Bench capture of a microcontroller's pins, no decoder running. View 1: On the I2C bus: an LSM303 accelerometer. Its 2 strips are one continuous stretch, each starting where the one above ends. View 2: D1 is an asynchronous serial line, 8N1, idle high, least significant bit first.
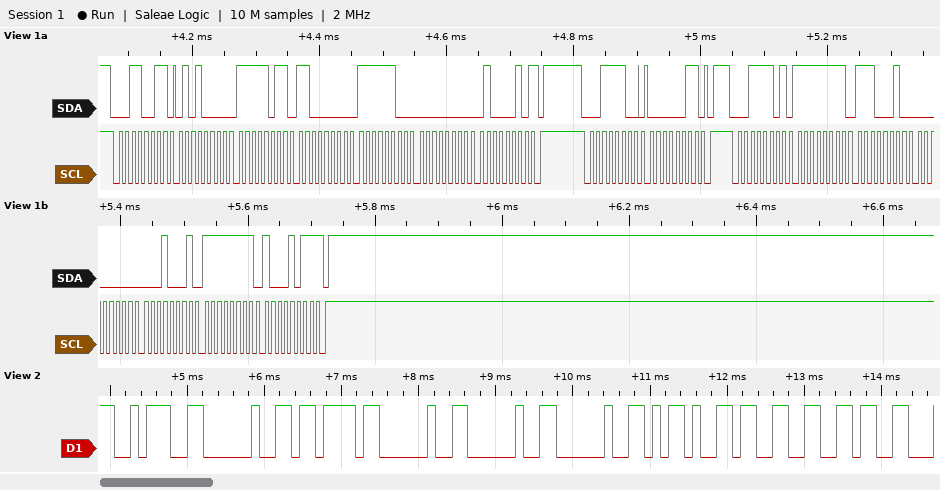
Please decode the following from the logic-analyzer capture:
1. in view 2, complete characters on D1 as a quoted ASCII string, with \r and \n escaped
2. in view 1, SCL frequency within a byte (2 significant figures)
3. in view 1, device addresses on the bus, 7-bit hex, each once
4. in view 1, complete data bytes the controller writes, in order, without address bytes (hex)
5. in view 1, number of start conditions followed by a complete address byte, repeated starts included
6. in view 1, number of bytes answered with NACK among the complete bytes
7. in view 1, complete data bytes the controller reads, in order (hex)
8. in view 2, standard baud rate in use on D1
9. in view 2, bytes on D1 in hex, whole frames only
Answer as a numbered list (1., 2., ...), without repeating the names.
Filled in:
1. ": {   -36"
2. 100 kHz
3. 0x19 0x1E
4. 03
5. 3
6. 2
7. 50 FB C0 FC 00 42 FF E2 00 11 FF 8B
8. 9600 baud
9. 3A 20 7B 20 20 20 2D 33 36
